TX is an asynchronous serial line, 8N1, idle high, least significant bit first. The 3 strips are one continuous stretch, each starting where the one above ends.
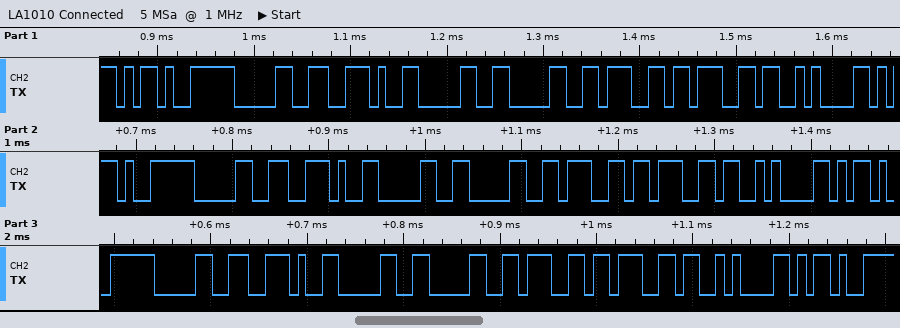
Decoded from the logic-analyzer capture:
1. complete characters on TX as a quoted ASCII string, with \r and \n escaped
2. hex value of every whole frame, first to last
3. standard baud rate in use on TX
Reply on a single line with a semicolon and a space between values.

"-0.00gg\n-0.00gg\n-0.00gg\n-"; 2D 30 2E 30 30 67 67 0A 2D 30 2E 30 30 67 67 0A 2D 30 2E 30 30 67 67 0A 2D; 115200 baud
